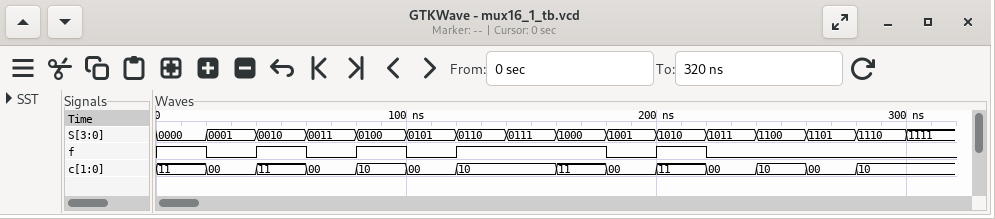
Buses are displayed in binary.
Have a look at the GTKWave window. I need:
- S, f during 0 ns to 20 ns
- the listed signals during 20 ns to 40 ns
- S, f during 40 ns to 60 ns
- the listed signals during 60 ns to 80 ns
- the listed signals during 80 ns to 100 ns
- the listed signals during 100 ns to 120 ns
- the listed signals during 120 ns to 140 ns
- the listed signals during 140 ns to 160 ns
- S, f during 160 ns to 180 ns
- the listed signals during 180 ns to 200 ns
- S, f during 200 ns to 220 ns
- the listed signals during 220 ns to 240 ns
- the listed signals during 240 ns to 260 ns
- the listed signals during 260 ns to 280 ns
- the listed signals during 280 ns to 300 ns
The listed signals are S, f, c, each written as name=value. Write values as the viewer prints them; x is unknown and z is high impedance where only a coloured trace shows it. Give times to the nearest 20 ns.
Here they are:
S=0000, f=1
S=0001, f=0, c=00
S=0010, f=1
S=0011, f=0, c=00
S=0100, f=1, c=10
S=0101, f=0, c=00
S=0110, f=1, c=10
S=0111, f=1, c=10
S=1000, f=1
S=1001, f=0, c=00
S=1010, f=1
S=1011, f=0, c=00
S=1100, f=0, c=10
S=1101, f=0, c=00
S=1110, f=0, c=10
